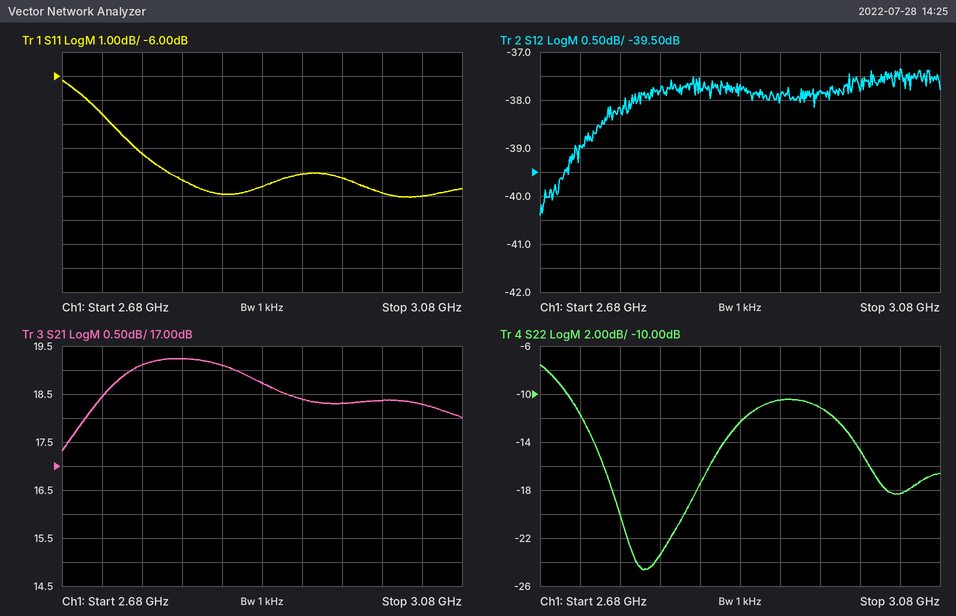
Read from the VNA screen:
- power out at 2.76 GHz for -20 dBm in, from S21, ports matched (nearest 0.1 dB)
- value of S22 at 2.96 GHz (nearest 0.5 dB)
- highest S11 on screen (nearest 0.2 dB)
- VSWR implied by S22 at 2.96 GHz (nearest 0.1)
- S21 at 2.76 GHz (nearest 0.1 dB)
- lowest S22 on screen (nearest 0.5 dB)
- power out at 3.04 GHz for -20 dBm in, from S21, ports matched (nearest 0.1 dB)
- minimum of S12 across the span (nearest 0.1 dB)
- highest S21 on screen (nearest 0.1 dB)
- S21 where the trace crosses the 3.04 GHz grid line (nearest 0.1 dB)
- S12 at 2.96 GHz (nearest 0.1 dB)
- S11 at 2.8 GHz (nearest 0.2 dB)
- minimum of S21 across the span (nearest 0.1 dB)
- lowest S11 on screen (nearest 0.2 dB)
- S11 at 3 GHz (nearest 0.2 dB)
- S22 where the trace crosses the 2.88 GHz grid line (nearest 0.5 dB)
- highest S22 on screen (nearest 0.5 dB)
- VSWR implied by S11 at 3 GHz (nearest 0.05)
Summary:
-0.9 dBm
-11.0 dB
-6.2 dB
1.8
19.1 dB
-24.5 dB
-1.7 dBm
-40.4 dB
19.2 dB
18.3 dB
-37.8 dB
-10.4 dB
17.3 dB
-11.0 dB
-10.8 dB
-12.5 dB
-7.5 dB
1.80
